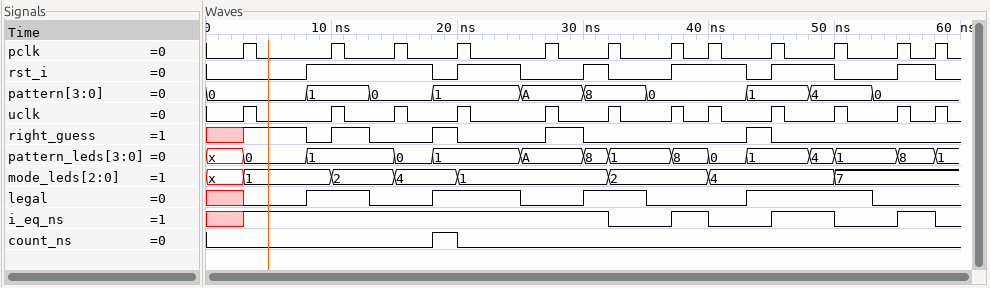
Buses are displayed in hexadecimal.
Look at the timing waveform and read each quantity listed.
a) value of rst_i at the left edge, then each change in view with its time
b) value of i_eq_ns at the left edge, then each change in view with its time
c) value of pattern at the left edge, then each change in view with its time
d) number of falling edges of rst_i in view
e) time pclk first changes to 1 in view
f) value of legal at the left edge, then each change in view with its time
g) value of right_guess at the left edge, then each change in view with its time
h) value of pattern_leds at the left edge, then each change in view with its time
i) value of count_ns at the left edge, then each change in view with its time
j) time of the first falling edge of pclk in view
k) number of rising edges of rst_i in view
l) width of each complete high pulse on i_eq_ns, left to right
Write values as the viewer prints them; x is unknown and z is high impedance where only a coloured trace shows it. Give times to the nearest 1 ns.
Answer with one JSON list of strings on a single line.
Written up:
["0, 1 at 8 ns, 0 at 18 ns, 1 at 20 ns, 0 at 25 ns, 1 at 30 ns, 0 at 32 ns, 1 at 37 ns, 0 at 43 ns, 1 at 45 ns, 0 at 50 ns, 1 at 55 ns, 0 at 58 ns", "x, 1 at 3 ns, 0 at 32 ns, 1 at 37 ns, 0 at 40 ns, 1 at 45 ns, 0 at 50 ns, 1 at 55 ns, 0 at 58 ns", "0, 1 at 8 ns, 0 at 13 ns, 1 at 18 ns, A at 25 ns, 8 at 30 ns, 0 at 35 ns, 1 at 43 ns, 4 at 48 ns, 0 at 53 ns", "6", "3 ns", "x, 0 at 3 ns, 1 at 8 ns, 0 at 13 ns, 1 at 18 ns, 0 at 25 ns, 1 at 30 ns, 0 at 35 ns, 1 at 43 ns, 0 at 53 ns", "x, 1 at 3 ns, 0 at 8 ns, 1 at 10 ns, 0 at 13 ns, 1 at 18 ns, 0 at 20 ns, 1 at 27 ns, 0 at 30 ns, 1 at 43 ns, 0 at 45 ns", "x, 0 at 3 ns, 1 at 8 ns, 0 at 15 ns, 1 at 18 ns, A at 25 ns, 8 at 30 ns, 1 at 32 ns, 8 at 37 ns, 0 at 40 ns, 1 at 43 ns, 4 at 48 ns, 1 at 50 ns, 8 at 55 ns, 1 at 58 ns", "0, 1 at 18 ns, 0 at 20 ns", "4 ns", "6", "3 ns, 5 ns, 3 ns"]
